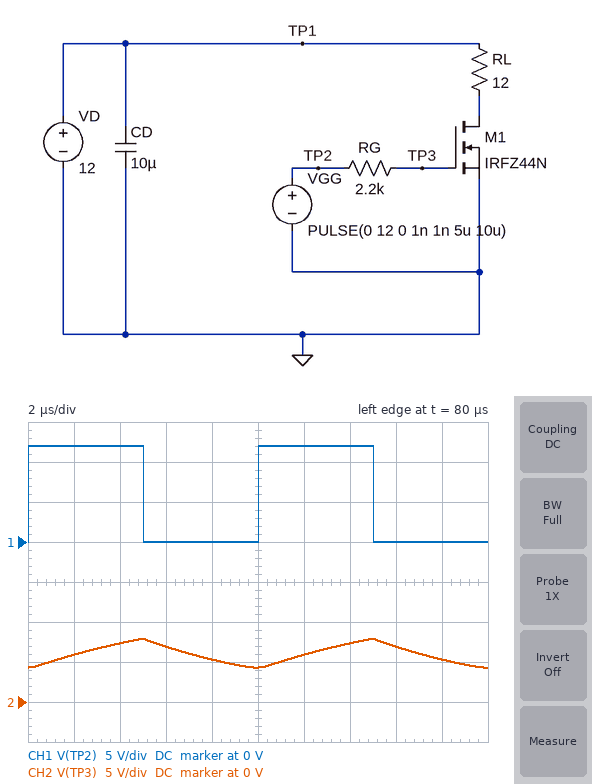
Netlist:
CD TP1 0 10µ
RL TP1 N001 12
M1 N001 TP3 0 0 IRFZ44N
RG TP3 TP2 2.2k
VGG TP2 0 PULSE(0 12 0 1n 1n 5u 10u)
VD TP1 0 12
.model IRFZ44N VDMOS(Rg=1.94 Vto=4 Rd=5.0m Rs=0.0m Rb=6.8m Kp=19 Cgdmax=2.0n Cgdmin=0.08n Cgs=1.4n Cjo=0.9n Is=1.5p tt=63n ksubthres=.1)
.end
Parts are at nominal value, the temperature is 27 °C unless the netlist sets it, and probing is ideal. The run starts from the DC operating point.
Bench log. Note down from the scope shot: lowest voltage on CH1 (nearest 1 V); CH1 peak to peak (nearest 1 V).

0 V
12 V
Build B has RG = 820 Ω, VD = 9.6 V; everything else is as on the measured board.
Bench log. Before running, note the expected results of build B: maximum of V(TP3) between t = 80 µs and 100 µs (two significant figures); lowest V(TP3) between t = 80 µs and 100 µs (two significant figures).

9.9 V
2.7 V
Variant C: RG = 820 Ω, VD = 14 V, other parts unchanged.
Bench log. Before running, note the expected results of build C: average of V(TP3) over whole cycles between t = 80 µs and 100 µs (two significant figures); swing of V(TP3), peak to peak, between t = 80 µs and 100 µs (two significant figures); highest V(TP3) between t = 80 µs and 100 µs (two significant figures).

6.0 V
7.0 V
9.9 V
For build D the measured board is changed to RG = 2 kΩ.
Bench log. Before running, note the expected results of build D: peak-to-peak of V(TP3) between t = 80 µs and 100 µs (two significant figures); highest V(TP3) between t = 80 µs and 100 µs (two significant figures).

3.8 V
8.1 V
